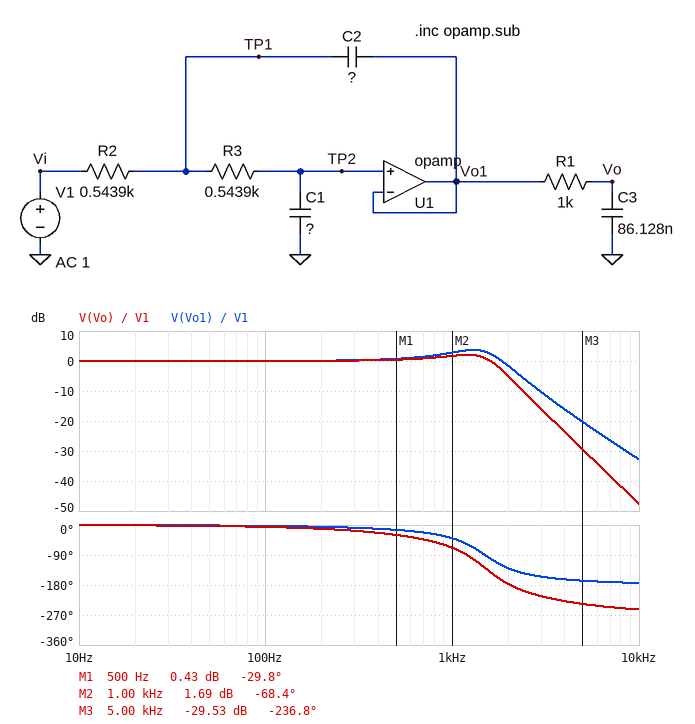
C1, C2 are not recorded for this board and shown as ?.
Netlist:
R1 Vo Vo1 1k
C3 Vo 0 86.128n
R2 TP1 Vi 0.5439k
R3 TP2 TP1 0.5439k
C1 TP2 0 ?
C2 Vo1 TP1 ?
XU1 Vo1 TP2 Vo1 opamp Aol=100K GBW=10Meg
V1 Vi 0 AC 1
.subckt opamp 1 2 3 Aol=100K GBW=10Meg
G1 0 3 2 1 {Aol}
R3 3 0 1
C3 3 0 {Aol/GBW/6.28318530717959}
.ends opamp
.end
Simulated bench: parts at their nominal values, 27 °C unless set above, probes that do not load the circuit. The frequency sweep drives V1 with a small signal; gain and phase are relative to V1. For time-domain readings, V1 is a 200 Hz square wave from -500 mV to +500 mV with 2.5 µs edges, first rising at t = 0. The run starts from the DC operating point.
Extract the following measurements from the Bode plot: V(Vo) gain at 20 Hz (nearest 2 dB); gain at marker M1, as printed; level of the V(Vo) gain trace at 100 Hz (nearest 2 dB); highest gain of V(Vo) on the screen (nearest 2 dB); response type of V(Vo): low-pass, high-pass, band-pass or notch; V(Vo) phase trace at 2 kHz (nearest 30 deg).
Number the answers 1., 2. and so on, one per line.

1. 0 dB
2. 0.43 dB
3. 0 dB
4. 2 dB
5. low-pass
6. -180 deg
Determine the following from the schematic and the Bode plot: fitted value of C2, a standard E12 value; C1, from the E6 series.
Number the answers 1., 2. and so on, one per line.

1. 560 nF
2. 68 nF
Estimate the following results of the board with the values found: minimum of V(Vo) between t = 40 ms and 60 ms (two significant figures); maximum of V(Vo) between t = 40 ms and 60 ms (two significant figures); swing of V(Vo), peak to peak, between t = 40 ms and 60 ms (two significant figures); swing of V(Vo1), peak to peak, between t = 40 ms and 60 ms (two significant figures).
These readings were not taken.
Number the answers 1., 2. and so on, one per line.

1. -720 mV
2. 720 mV
3. 1.4 V
4. 1.6 V
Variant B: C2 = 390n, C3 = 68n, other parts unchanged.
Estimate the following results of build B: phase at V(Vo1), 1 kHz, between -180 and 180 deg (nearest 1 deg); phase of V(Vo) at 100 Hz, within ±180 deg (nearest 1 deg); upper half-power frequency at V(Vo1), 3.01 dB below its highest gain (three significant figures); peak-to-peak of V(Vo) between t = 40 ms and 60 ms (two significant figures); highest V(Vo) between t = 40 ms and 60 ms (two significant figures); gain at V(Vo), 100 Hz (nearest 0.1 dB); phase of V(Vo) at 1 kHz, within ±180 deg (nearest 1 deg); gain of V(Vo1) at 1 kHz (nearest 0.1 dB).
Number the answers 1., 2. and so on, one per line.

1. -34 deg
2. -5 deg
3. 2.13 kHz
4. 1.3 V
5. 670 mV
6. 0 dB
7. -57 deg
8. 1.6 dB
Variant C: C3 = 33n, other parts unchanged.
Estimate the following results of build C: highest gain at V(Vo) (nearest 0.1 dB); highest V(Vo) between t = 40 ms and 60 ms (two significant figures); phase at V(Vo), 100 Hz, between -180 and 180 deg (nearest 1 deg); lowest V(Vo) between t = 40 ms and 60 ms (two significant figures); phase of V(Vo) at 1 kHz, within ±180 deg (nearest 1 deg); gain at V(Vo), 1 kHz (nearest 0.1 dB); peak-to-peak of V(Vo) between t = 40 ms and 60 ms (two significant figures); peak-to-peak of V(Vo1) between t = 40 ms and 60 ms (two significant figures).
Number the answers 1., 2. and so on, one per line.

1. 3.4 dB
2. 800 mV
3. -4 deg
4. -800 mV
5. -52 deg
6. 2.6 dB
7. 1.6 V
8. 1.6 V
